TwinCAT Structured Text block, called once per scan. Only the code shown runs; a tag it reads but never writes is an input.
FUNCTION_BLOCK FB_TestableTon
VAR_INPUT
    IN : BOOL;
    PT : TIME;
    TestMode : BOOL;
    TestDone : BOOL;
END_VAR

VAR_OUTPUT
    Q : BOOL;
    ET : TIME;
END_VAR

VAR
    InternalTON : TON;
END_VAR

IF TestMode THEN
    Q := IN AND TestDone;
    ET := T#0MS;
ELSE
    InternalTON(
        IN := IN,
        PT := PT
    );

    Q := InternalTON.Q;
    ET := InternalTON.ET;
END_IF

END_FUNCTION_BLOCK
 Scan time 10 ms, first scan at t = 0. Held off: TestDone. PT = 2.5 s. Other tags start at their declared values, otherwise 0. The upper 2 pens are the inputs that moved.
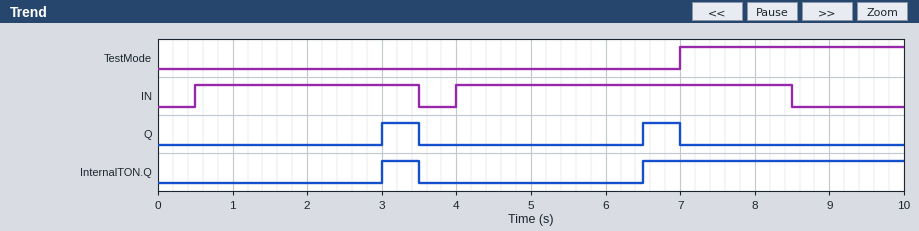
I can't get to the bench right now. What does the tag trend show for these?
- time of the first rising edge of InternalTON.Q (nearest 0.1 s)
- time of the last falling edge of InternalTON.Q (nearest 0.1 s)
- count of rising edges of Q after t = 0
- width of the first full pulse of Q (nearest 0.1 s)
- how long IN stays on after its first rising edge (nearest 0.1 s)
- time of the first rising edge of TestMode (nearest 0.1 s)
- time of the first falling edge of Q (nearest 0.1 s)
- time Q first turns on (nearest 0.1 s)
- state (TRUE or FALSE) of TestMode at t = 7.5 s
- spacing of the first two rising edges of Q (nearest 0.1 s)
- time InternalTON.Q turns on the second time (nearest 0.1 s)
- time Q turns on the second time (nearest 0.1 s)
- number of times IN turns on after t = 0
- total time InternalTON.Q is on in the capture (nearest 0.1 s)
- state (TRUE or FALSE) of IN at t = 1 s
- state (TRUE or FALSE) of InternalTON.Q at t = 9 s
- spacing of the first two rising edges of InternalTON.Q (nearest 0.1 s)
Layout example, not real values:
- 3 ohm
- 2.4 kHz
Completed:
- 3.0 s
- 3.5 s
- 2
- 0.5 s
- 3.0 s
- 7.0 s
- 3.5 s
- 3.0 s
- TRUE
- 3.5 s
- 6.5 s
- 6.5 s
- 2
- 4.0 s
- TRUE
- TRUE
- 3.5 s
